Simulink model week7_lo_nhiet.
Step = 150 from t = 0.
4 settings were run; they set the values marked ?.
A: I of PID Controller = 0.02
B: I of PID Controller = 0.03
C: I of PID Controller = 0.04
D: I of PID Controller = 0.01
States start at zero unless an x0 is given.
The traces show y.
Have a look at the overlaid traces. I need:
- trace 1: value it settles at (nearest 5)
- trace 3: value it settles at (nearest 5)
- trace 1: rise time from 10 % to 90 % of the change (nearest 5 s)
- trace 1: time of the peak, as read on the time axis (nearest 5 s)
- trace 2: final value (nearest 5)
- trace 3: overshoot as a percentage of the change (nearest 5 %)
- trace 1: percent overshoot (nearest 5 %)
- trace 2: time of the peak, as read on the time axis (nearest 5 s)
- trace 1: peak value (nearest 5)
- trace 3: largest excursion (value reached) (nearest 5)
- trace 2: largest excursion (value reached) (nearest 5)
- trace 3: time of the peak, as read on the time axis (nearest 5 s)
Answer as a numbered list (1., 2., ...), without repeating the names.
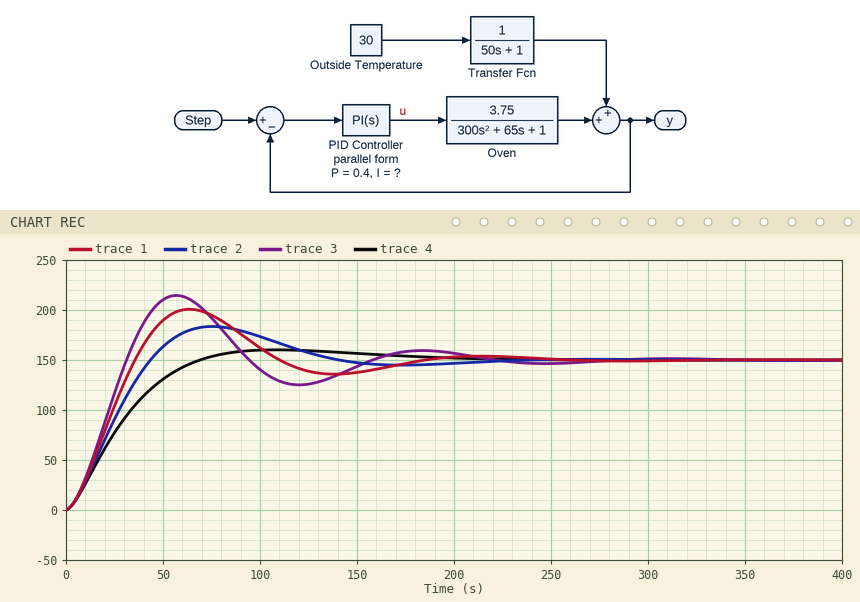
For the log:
1. 150
2. 150
3. 25 s
4. 65 s
5. 150
6. 45 %
7. 35 %
8. 75 s
9. 200
10. 215
11. 185
12. 55 s
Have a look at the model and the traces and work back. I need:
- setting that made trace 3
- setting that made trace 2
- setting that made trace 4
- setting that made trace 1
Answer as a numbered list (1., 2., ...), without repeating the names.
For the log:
1. C
2. A
3. D
4. B
